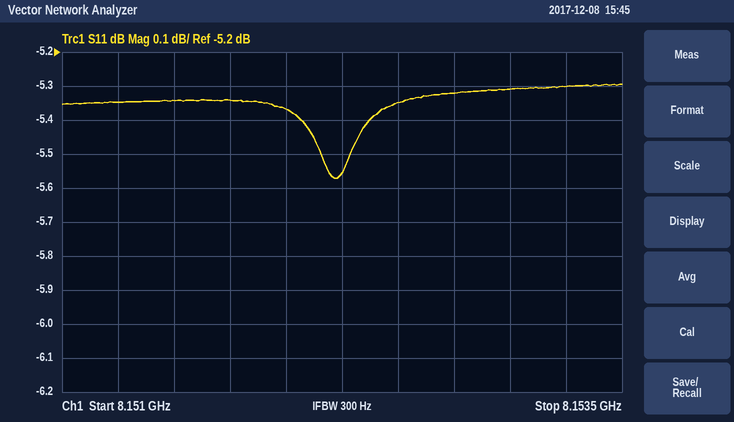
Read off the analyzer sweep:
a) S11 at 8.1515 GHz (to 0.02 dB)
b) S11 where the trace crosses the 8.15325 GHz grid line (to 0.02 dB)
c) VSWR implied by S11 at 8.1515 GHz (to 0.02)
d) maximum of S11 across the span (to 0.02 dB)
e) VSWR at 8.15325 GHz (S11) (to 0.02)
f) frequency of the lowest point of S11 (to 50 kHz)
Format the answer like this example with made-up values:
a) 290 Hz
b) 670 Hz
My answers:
a) -5.34 dB
b) -5.30 dB
c) 3.36
d) -5.30 dB
e) 3.38
f) 8.15220 GHz
